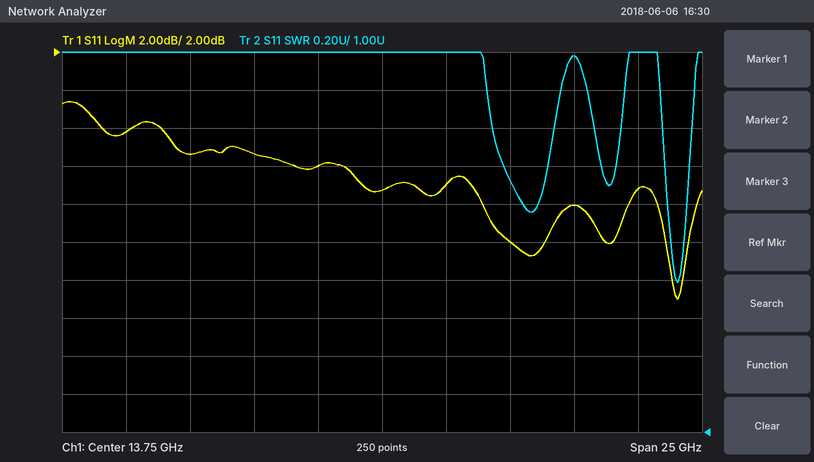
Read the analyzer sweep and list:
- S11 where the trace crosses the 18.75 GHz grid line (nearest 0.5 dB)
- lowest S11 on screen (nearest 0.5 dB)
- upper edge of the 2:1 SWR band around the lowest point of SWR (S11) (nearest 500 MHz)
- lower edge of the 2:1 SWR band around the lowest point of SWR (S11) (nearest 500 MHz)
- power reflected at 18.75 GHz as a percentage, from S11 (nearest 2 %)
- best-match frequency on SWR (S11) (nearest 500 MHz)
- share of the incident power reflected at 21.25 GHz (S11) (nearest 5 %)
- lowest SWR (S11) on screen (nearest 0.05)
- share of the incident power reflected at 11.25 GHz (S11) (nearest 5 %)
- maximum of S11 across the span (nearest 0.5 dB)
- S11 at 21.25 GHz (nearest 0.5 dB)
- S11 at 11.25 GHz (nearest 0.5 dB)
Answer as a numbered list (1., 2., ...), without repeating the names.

1. -8.0 dB
2. -11.0 dB
3. 25.5 GHz
4. 25.0 GHz
5. 16 %
6. 25.5 GHz
7. 25 %
8. 1.80
9. 40 %
10. -0.5 dB
11. -6.0 dB
12. -4.0 dB
